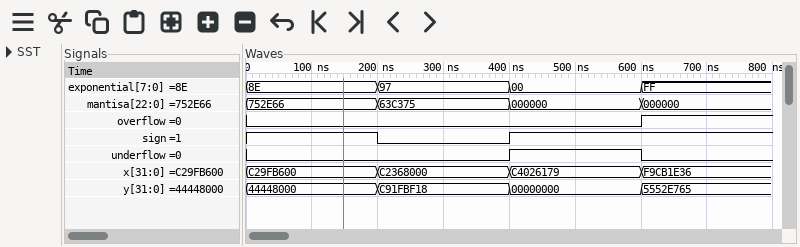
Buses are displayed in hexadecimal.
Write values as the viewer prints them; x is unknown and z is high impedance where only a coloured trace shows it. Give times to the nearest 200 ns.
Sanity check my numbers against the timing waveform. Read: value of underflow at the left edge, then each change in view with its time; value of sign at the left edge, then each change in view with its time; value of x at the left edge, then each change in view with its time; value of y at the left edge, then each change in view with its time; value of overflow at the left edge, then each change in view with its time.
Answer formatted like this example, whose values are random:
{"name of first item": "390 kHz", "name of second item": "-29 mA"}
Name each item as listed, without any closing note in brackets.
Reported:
{"value of underflow at the left edge, then each change in view with its time": "0, 1 at 400 ns, 0 at 600 ns", "value of sign at the left edge, then each change in view with its time": "1, 0 at 200 ns, 1 at 400 ns", "value of x at the left edge, then each change in view with its time": "C29FB600, C2368000 at 200 ns, C4026179 at 400 ns, F9CB1E36 at 600 ns", "value of y at the left edge, then each change in view with its time": "44448000, C91FBF18 at 200 ns, 00000000 at 400 ns, 5552E765 at 600 ns", "value of overflow at the left edge, then each change in view with its time": "0, 1 at 600 ns"}
